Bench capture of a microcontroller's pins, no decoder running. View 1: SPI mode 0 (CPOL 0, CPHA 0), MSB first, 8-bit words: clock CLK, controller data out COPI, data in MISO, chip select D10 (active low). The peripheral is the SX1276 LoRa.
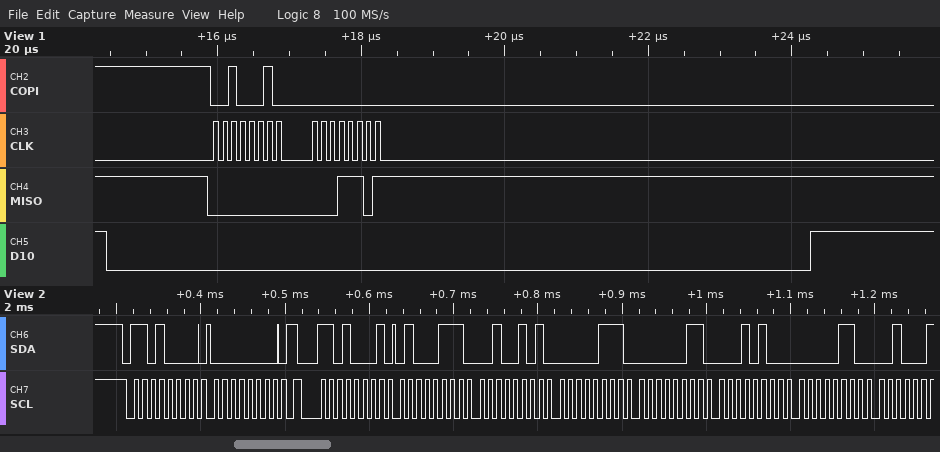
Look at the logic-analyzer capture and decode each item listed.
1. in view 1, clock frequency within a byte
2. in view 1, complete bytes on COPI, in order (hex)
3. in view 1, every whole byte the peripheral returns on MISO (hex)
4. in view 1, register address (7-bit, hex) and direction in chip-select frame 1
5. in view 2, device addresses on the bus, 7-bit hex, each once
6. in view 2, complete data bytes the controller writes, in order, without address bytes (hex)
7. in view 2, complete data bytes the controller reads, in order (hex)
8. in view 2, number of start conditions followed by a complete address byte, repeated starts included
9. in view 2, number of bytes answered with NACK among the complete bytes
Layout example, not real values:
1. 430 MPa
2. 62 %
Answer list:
1. 8 MHz
2. 0x22 0x00
3. 0x00 0x1D
4. 0x22 read
5. 0x68
6. 00
7. 47 25 07 03 14 06
8. 2
9. 0
